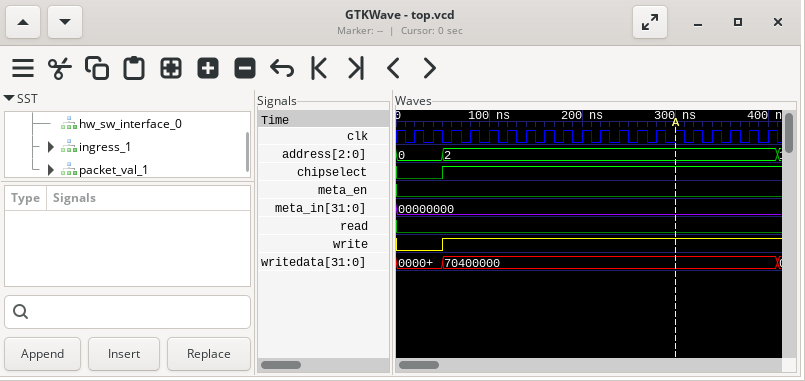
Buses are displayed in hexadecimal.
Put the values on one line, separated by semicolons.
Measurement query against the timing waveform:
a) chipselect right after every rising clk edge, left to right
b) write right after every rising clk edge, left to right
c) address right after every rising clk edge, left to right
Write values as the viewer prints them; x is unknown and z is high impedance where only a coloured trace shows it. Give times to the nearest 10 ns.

0 0 1 1 1 1 1 1 1 1 1 1 1 1 1 1 1 1 1 1; 0 0 1 1 1 1 1 1 1 1 1 1 1 1 1 1 1 1 1 1; 0, 0, 2, 2, 2, 2, 2, 2, 2, 2, 2, 2, 2, 2, 2, 2, 2, 2, 2, 2
